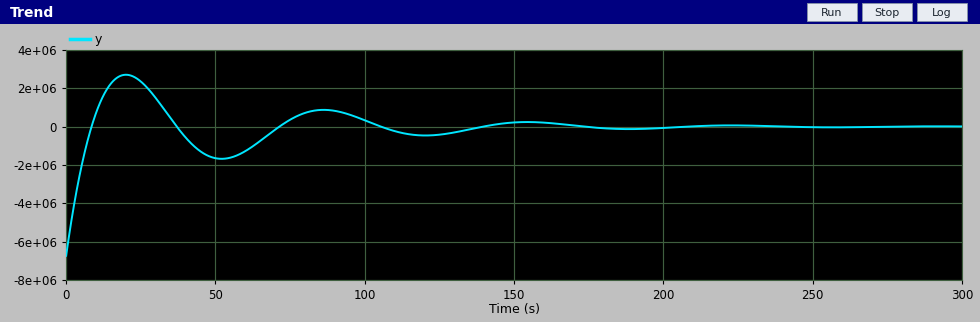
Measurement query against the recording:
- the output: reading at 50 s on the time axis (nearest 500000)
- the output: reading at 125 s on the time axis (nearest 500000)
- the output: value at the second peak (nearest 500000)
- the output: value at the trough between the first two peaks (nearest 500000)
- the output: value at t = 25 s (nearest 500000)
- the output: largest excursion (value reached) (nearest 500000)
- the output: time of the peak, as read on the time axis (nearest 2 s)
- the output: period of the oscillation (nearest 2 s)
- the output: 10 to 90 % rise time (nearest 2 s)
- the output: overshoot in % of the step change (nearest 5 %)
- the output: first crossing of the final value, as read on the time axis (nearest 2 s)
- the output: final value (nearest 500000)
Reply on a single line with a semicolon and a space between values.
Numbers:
-1500000; -500000; 1000000; -1500000; 2500000; 2500000; 20 s; 66 s; 6 s; 40 %; 8 s; 0
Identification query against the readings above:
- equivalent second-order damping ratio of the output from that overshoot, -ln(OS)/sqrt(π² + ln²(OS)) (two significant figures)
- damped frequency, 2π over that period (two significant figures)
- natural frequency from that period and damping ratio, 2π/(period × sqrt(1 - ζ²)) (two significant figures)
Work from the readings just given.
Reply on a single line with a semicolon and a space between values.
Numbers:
0.28; 0.095 rad/s; 0.099 rad/s
